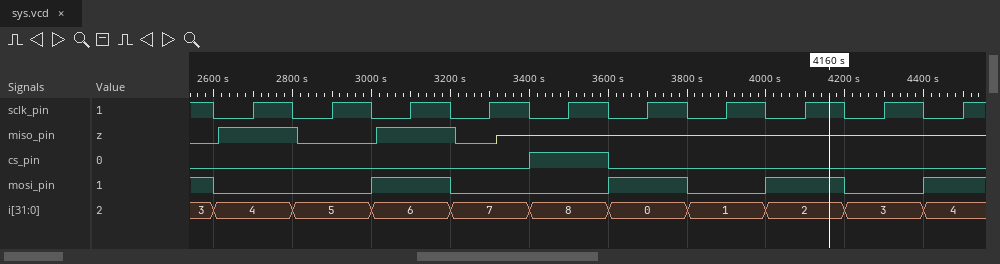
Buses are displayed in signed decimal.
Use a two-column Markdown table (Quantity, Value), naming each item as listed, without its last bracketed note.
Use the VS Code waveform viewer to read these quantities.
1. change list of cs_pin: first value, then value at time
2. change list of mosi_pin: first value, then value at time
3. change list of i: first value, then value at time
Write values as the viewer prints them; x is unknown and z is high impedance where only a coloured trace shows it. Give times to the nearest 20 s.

| Quantity | Value |
|---|---|
| change list of cs_pin: first value, then value at time | 0, 1 at 3400 s, 0 at 3600 s |
| change list of mosi_pin: first value, then value at time | 1, 0 at 2600 s, 1 at 3000 s, 0 at 3200 s, 1 at 3600 s, 0 at 3800 s, 1 at 4000 s, 0 at 4200 s, 1 at 4400 s |
| change list of i: first value, then value at time | 3, 4 at 2600 s, 5 at 2800 s, 6 at 3000 s, 7 at 3200 s, 8 at 3400 s, 0 at 3600 s, 1 at 3800 s, 2 at 4000 s, 3 at 4200 s, 4 at 4400 s |
